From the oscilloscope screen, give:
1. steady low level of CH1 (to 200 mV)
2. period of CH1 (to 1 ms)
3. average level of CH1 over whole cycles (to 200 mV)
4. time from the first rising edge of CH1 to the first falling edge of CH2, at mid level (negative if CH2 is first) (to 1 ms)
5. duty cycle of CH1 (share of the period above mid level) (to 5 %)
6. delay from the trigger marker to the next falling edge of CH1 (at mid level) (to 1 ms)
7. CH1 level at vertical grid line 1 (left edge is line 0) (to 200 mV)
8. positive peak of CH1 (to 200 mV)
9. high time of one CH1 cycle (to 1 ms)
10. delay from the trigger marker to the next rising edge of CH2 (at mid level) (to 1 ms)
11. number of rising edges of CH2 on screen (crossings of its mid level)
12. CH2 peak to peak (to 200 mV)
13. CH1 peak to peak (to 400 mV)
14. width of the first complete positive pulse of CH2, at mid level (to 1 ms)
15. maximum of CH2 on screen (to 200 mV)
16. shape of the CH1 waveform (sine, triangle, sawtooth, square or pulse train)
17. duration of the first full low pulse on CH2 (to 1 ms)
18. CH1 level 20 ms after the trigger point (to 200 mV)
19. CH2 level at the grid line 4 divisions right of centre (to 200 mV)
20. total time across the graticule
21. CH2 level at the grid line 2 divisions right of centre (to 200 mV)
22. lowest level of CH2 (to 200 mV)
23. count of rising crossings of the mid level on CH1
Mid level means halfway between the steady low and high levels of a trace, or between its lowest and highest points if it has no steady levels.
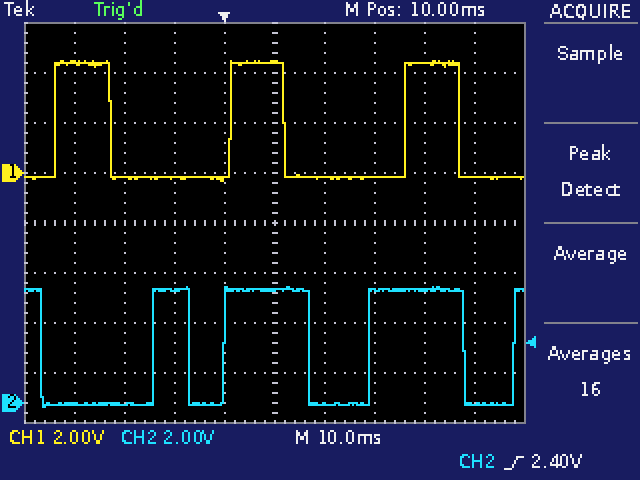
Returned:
-200 mV
35 ms
1.2 V
-3 ms
30 %
12 ms
4.4 V
4.4 V
11 ms
29 ms
4
4.8 V
4.8 V
7 ms
4.6 V
pulse train
22 ms
-200 mV
0.0 V
100 ms
4.6 V
-200 mV
3
